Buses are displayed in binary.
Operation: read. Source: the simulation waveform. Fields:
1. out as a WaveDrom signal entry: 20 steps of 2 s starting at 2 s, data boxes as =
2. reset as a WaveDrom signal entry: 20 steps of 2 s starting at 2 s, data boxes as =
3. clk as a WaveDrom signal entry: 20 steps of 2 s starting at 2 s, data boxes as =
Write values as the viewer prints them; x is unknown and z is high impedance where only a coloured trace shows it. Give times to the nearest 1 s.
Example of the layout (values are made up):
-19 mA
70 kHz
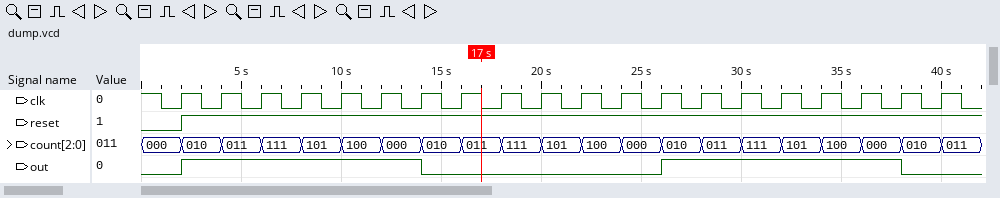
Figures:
{name: 'out', wave: '1.....0.....1.....0.'}
{name: 'reset', wave: '1...................'}
{name: 'clk', wave: 'p...................'}
